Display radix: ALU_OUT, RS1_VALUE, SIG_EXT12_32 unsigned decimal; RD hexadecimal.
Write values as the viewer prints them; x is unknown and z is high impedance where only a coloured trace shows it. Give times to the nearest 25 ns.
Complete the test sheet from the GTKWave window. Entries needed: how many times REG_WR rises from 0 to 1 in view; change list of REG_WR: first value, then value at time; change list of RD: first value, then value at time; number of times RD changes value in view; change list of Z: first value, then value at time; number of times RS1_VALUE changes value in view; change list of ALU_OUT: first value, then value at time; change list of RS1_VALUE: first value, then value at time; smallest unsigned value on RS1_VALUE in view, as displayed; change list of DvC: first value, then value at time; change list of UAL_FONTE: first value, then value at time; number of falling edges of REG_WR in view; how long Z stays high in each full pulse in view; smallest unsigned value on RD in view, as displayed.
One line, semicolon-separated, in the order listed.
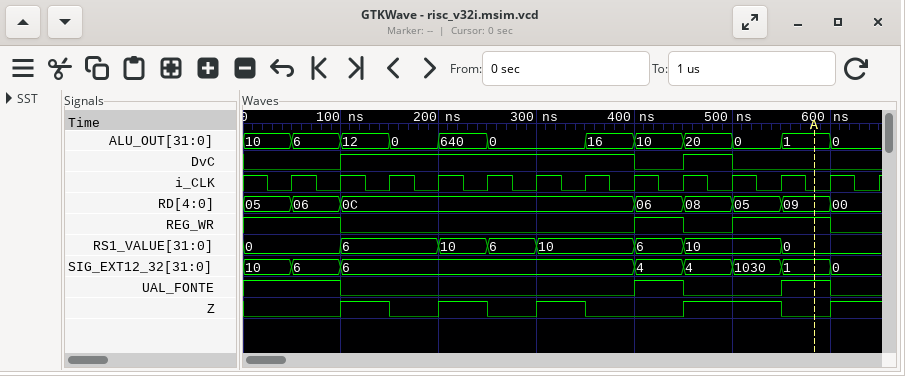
2; 1, 0 at 100 ns, 1 at 400 ns, 0 at 450 ns, 1 at 500 ns, 0 at 600 ns; 05, 06 at 50 ns, 0C at 100 ns, 06 at 400 ns, 08 at 450 ns, 05 at 500 ns, 09 at 550 ns, 00 at 600 ns; 7; 0, 1 at 100 ns, 0 at 150 ns, 1 at 200 ns, 0 at 250 ns, 1 at 300 ns, 0 at 350 ns, 1 at 450 ns, 0 at 550 ns, 1 at 600 ns; 7; 10, 6 at 50 ns, 12 at 100 ns, 0 at 150 ns, 640 at 200 ns, 0 at 250 ns, 16 at 350 ns, 10 at 400 ns, 20 at 450 ns, 0 at 500 ns, 1 at 550 ns, 0 at 600 ns; 0, 6 at 100 ns, 10 at 200 ns, 6 at 250 ns, 10 at 300 ns, 6 at 400 ns, 10 at 450 ns, 0 at 550 ns; 0; 0, 1 at 100 ns, 0 at 400 ns, 1 at 450 ns, 0 at 500 ns; 1, 0 at 100 ns, 1 at 400 ns, 0 at 450 ns, 1 at 550 ns, 0 at 600 ns; 3; 50 ns, 50 ns, 50 ns, 100 ns; 00
